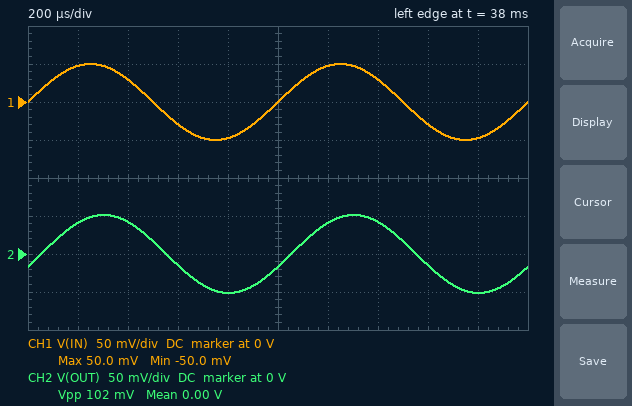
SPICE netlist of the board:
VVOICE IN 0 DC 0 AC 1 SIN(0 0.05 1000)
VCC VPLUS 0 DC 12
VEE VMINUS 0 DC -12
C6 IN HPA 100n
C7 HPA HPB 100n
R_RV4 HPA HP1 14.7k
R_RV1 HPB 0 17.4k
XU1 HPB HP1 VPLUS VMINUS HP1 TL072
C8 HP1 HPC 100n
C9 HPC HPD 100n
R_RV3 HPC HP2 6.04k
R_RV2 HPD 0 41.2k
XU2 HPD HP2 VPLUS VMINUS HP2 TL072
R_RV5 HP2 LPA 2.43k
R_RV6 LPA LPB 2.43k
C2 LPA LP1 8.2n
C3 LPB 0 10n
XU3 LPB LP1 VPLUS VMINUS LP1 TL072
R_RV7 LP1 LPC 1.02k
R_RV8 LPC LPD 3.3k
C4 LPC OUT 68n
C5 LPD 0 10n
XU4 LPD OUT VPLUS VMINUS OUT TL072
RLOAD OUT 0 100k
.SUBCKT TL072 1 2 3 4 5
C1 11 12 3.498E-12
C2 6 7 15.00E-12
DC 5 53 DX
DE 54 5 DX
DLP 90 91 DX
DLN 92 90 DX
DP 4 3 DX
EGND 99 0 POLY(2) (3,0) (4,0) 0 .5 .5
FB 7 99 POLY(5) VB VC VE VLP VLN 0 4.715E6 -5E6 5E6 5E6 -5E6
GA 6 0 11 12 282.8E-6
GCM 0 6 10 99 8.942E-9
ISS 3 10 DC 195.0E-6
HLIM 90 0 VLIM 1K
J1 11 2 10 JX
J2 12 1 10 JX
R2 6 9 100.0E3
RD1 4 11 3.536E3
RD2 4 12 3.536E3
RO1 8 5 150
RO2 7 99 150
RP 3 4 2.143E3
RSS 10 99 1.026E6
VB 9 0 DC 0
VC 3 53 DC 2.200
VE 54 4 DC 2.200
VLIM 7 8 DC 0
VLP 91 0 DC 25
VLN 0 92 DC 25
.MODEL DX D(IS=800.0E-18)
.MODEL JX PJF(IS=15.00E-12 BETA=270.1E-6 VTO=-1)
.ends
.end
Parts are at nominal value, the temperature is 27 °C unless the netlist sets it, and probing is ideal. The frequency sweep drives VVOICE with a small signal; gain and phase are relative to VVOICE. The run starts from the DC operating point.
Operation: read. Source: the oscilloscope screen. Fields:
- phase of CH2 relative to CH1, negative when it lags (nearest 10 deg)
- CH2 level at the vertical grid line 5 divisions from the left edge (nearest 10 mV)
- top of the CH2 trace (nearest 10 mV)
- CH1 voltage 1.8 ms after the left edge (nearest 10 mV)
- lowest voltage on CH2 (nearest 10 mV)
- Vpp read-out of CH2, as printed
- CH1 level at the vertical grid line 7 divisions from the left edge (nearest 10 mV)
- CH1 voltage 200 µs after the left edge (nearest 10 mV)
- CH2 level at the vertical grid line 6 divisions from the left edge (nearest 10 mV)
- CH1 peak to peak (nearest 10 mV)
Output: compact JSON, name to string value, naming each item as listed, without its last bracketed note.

{"phase of CH2 relative to CH1, negative when it lags": "-20 deg", "CH2 level at the vertical grid line 5 divisions from the left edge": "-20 mV", "top of the CH2 trace": "50 mV", "CH1 voltage 1.8 ms after the left edge": "-50 mV", "lowest voltage on CH2": "-50 mV", "Vpp read-out of CH2, as printed": "102 mV", "CH1 level at the vertical grid line 7 divisions from the left edge": "30 mV", "CH1 voltage 200 µs after the left edge": "50 mV", "CH2 level at the vertical grid line 6 divisions from the left edge": "40 mV", "CH1 peak to peak": "100 mV"}
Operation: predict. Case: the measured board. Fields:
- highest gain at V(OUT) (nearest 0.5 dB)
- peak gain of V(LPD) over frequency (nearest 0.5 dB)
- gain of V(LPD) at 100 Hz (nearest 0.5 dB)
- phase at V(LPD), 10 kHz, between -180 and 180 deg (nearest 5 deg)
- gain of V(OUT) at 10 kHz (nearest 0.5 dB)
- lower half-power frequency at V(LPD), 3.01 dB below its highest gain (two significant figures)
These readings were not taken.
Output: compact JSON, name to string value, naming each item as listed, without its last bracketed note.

{"highest gain at V(OUT)": "0.5 dB", "peak gain of V(LPD) over frequency": "0.5 dB", "gain of V(LPD) at 100 Hz": "-3.0 dB", "phase at V(LPD), 10 kHz, between -180 and 180 deg": "95 deg", "gain of V(OUT) at 10 kHz": "-28.5 dB", "lower half-power frequency at V(LPD), 3.01 dB below its highest gain": "100 Hz"}
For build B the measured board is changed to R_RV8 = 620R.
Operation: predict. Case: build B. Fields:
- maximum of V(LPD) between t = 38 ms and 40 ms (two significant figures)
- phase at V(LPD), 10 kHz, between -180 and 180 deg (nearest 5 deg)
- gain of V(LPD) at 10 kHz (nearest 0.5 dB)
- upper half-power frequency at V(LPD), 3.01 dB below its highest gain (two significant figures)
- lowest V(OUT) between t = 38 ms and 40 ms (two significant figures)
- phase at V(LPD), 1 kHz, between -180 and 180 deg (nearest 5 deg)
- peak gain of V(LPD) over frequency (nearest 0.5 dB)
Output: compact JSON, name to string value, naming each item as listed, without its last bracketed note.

{"maximum of V(LPD) between t = 38 ms and 40 ms": "49 mV", "phase at V(LPD), 10 kHz, between -180 and 180 deg": "130 deg", "gain of V(LPD) at 10 kHz": "-12.0 dB", "upper half-power frequency at V(LPD), 3.01 dB below its highest gain": "6.3 kHz", "lowest V(OUT) between t = 38 ms and 40 ms": "-49 mV", "phase at V(LPD), 1 kHz, between -180 and 180 deg": "-10 deg", "peak gain of V(LPD) over frequency": "0 dB"}
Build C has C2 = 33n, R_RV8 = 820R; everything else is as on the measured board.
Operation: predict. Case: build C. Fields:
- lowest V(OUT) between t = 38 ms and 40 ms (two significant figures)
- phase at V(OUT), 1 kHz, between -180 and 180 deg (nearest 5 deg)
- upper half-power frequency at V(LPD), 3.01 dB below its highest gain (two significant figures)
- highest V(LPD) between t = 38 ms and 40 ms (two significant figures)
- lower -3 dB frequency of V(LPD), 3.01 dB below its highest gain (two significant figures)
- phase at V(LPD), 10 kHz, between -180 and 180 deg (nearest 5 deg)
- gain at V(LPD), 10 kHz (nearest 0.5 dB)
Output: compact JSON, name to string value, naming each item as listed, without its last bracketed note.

{"lowest V(OUT) between t = 38 ms and 40 ms": "-52 mV", "phase at V(OUT), 1 kHz, between -180 and 180 deg": "-10 deg", "upper half-power frequency at V(LPD), 3.01 dB below its highest gain": "4.7 kHz", "highest V(LPD) between t = 38 ms and 40 ms": "52 mV", "lower -3 dB frequency of V(LPD), 3.01 dB below its highest gain": "110 Hz", "phase at V(LPD), 10 kHz, between -180 and 180 deg": "70 deg", "gain at V(LPD), 10 kHz": "-22.0 dB"}
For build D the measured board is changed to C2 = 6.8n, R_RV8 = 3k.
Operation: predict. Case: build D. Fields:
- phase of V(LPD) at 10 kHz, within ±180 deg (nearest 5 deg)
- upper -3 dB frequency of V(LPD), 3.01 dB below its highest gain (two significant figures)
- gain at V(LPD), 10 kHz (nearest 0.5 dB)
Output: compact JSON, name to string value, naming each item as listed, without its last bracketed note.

{"phase of V(LPD) at 10 kHz, within ±180 deg": "100 deg", "upper -3 dB frequency of V(LPD), 3.01 dB below its highest gain": "3.7 kHz", "gain at V(LPD), 10 kHz": "-27.5 dB"}
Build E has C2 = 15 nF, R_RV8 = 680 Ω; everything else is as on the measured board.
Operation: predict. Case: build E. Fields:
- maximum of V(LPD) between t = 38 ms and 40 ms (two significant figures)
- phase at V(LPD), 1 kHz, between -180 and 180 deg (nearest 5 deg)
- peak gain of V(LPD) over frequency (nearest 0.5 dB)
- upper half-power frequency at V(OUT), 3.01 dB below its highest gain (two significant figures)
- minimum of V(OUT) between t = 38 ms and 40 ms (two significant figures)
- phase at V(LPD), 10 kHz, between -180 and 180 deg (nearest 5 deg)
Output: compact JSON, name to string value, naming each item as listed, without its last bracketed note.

{"maximum of V(LPD) between t = 38 ms and 40 ms": "50 mV", "phase at V(LPD), 1 kHz, between -180 and 180 deg": "-10 deg", "peak gain of V(LPD) over frequency": "0 dB", "upper half-power frequency at V(OUT), 3.01 dB below its highest gain": "6.3 kHz", "minimum of V(OUT) between t = 38 ms and 40 ms": "-50 mV", "phase at V(LPD), 10 kHz, between -180 and 180 deg": "100 deg"}
